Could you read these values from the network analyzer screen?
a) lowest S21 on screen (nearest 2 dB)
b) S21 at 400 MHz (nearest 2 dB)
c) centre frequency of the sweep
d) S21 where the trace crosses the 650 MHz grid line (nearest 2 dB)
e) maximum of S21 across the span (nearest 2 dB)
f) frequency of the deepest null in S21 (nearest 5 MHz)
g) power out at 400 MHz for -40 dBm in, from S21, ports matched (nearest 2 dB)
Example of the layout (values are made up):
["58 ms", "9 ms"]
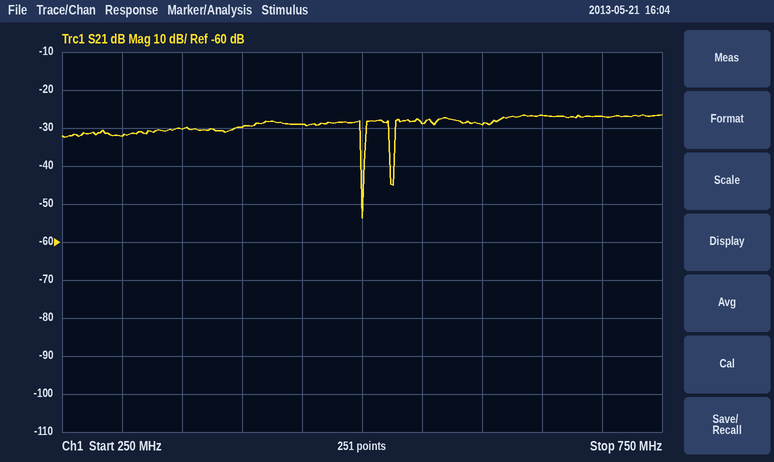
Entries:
["-54 dB", "-30 dB", "500 MHz", "-26 dB", "-26 dB", "500 MHz", "-70 dBm"]
